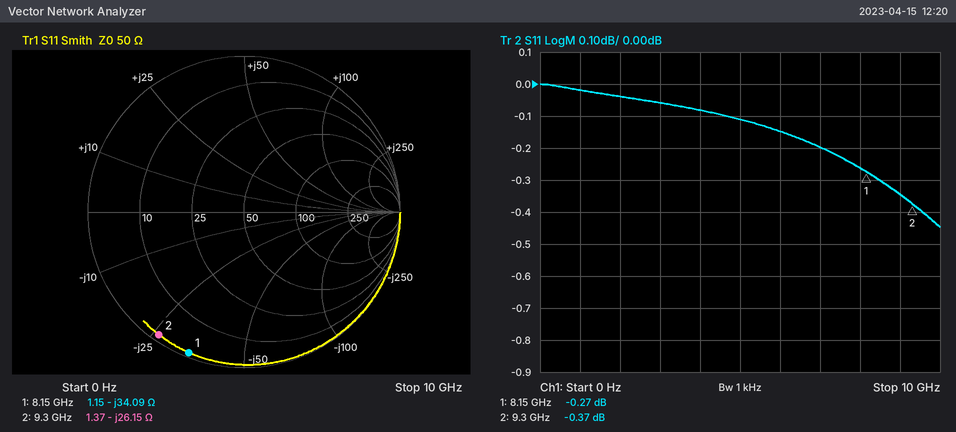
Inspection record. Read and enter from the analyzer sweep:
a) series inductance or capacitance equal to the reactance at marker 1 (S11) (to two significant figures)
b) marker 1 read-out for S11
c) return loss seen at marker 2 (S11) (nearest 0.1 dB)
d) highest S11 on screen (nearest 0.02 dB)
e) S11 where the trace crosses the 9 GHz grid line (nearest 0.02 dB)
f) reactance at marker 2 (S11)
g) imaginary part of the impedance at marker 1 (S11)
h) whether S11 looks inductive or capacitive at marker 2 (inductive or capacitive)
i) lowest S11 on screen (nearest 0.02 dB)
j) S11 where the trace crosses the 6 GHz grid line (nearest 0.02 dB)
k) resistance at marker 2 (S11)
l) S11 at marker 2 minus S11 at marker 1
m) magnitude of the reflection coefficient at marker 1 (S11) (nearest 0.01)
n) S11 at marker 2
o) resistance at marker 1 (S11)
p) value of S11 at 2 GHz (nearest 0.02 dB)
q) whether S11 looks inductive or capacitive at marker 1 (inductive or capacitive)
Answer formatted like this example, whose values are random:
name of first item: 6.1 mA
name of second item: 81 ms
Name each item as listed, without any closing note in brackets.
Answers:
series inductance or capacitance equal to the reactance at marker 1 (S11): 570 fF
marker 1 read-out for S11: -0.27 dB
return loss seen at marker 2 (S11): 0.4 dB
highest S11 on screen: 0.00 dB
S11 where the trace crosses the 9 GHz grid line: -0.34 dB
reactance at marker 2: -26.15 Ω
imaginary part of the impedance at marker 1: -34.09 Ω
whether S11 looks inductive or capacitive at marker 2: capacitive
lowest S11 on screen: -0.44 dB
S11 where the trace crosses the 6 GHz grid line: -0.14 dB
resistance at marker 2: 1.37 Ω
S11 at marker 2 minus S11 at marker 1: -0.10 dB
magnitude of the reflection coefficient at marker 1 (S11): 0.97
S11 at marker 2: -0.37 dB
resistance at marker 1: 1.15 Ω
value of S11 at 2 GHz: -0.04 dB
whether S11 looks inductive or capacitive at marker 1: capacitive
